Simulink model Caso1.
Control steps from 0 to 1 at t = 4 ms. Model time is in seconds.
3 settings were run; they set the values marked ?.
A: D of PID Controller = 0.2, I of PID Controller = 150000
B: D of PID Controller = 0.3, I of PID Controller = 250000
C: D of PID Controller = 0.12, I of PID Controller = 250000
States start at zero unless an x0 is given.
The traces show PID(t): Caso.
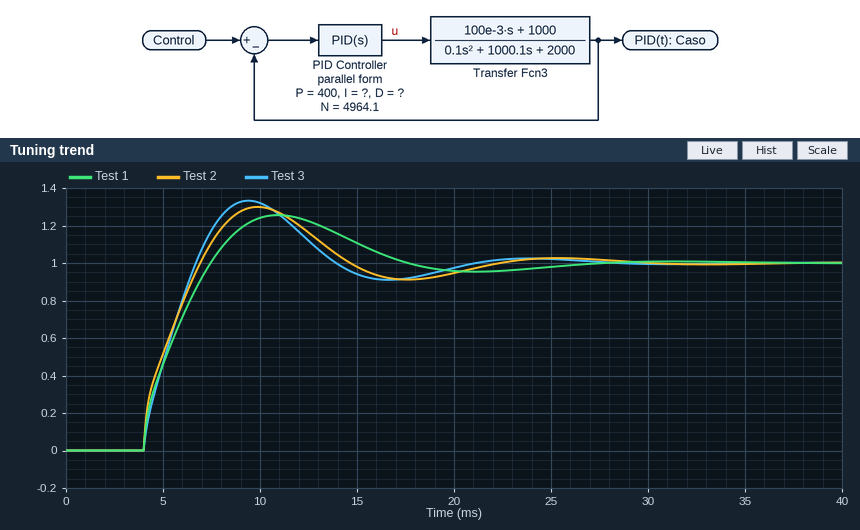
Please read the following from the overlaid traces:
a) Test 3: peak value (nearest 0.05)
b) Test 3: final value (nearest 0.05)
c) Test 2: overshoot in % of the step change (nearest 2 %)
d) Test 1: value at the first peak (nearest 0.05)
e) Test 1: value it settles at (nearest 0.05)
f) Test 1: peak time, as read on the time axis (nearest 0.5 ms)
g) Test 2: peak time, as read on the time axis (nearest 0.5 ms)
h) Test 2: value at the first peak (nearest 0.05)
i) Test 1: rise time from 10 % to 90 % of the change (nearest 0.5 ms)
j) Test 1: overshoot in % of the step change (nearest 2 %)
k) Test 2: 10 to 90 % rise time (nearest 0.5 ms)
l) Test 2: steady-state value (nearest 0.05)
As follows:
1.35
1.00
30 %
1.25
1.00
11.0 ms
10.0 ms
1.30
3.0 ms
26 %
2.5 ms
1.00
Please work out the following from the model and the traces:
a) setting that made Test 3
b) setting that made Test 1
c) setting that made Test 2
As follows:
C
A
B
